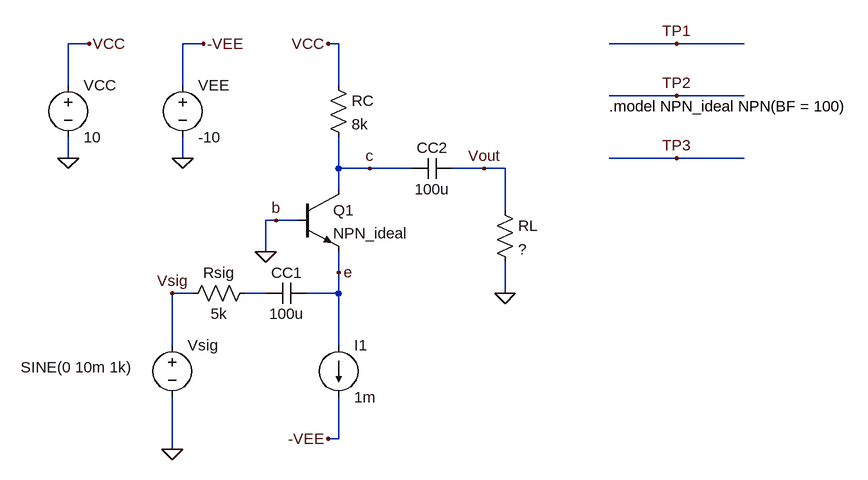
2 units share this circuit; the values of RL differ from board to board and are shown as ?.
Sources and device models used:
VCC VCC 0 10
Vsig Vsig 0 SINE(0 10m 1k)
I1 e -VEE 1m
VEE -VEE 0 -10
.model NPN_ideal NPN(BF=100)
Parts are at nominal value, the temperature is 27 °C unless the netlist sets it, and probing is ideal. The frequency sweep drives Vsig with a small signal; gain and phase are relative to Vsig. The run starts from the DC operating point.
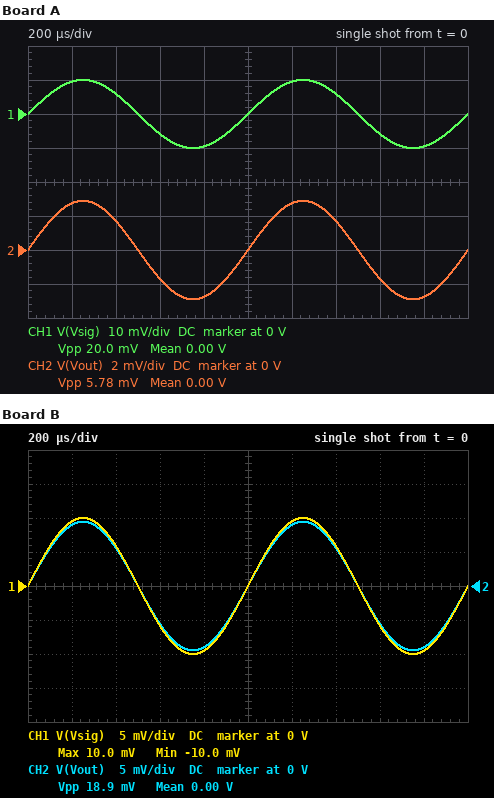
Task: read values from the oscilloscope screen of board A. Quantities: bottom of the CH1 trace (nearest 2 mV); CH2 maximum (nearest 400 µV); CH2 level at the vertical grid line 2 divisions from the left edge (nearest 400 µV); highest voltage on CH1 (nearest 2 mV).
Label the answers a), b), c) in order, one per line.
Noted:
a) -10 mV
b) 2.8 mV
c) 1.6 mV
d) 10 mV
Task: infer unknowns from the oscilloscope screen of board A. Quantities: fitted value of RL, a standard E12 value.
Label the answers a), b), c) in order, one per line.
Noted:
a) 1.8 kΩ
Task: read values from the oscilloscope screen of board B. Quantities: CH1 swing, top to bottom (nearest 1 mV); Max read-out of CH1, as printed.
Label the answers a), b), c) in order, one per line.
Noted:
a) 20 mV
b) 10.0 mV
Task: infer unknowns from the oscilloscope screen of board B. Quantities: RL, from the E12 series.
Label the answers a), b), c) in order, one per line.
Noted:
a) 12 kΩ
